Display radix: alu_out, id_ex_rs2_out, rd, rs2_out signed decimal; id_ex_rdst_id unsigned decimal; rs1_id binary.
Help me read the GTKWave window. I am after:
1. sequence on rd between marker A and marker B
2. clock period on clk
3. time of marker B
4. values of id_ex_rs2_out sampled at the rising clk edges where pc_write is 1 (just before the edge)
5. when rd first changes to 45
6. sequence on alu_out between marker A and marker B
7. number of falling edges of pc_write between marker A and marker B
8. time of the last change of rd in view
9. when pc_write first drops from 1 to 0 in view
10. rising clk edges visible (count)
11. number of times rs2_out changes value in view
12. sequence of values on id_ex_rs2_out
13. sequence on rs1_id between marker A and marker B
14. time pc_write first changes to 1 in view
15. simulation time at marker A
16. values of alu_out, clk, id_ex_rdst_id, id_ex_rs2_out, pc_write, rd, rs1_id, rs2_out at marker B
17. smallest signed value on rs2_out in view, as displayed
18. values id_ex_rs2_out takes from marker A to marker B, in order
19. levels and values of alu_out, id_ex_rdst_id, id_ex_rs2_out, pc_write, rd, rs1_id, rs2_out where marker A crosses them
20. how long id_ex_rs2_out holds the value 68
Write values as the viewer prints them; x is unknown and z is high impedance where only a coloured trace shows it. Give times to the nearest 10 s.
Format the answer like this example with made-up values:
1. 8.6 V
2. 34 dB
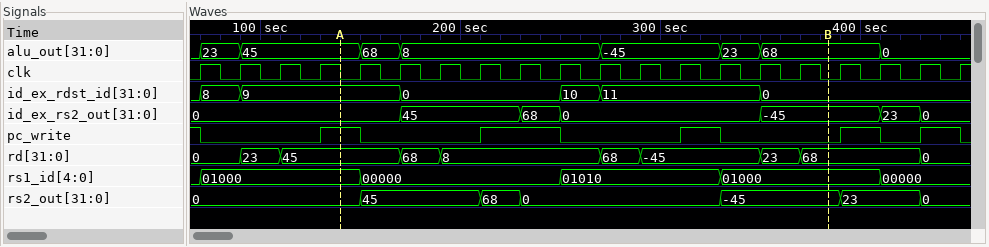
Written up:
1. 45, 68, 8, 68, -45, 23, 68
2. 20 s
3. 380 s
4. 0, 0, 45, 68, 0, -45, 0
5. 110 s
6. 45, 68, 8, -45, 23, 68
7. 3
8. 430 s
9. 70 s
10. 20
11. 6
12. 0, 45, 68, 0, -45, 23, 0
13. 01000, 00000, 01010, 01000
14. 130 s
15. 140 s
16. alu_out=68, clk=0, id_ex_rdst_id=0, id_ex_rs2_out=-45, pc_write=0, rd=68, rs1_id=01000, rs2_out=-45
17. -45
18. 0, 45, 68, 0, -45
19. alu_out=45, id_ex_rdst_id=9, id_ex_rs2_out=0, pc_write=1, rd=45, rs1_id=01000, rs2_out=0
20. 20 s
